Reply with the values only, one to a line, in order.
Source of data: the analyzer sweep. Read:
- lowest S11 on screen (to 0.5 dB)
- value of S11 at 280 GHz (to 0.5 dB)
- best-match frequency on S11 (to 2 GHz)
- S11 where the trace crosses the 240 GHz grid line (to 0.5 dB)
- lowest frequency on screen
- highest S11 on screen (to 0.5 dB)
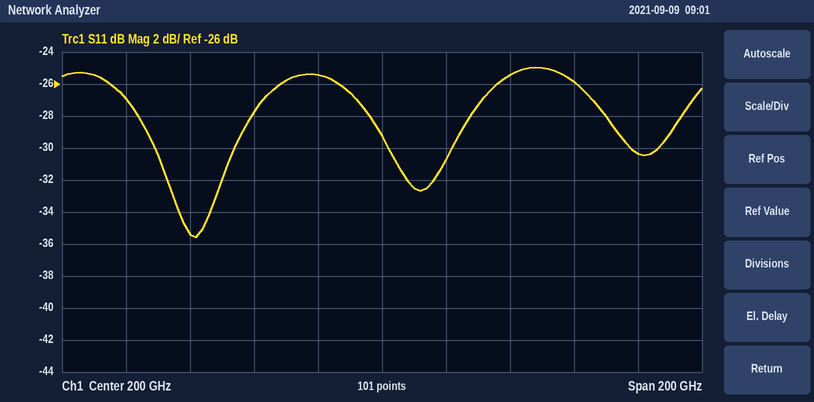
-35.5 dB
-30.5 dB
142 GHz
-25.5 dB
100 GHz
-25.0 dB
